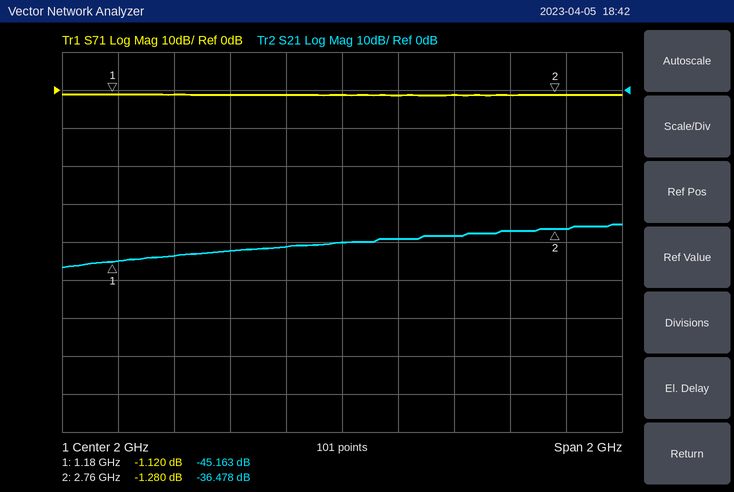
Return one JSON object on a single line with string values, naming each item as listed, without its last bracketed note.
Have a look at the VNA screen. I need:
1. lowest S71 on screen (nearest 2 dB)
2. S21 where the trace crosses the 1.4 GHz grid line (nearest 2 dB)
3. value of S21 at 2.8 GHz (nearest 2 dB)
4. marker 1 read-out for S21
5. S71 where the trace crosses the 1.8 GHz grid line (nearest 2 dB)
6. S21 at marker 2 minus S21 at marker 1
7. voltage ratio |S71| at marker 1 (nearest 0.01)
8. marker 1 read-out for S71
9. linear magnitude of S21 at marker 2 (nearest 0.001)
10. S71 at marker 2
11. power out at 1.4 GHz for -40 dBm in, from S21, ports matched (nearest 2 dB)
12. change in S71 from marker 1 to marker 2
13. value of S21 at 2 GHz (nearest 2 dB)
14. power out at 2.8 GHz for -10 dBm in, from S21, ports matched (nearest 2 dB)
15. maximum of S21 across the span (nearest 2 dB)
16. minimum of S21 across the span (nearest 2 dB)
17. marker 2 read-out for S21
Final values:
{"lowest S71 on screen": "-2 dB", "S21 where the trace crosses the 1.4 GHz grid line": "-44 dB", "value of S21 at 2.8 GHz": "-36 dB", "marker 1 read-out for S21": "-45.163 dB", "S71 where the trace crosses the 1.8 GHz grid line": "-2 dB", "S21 at marker 2 minus S21 at marker 1": "8.685 dB", "voltage ratio |S71| at marker 1": "0.88", "marker 1 read-out for S71": "-1.120 dB", "linear magnitude of S21 at marker 2": "0.015", "S71 at marker 2": "-1.280 dB", "power out at 1.4 GHz for -40 dBm in, from S21, ports matched": "-84 dBm", "change in S71 from marker 1 to marker 2": "-0.160 dB", "value of S21 at 2 GHz": "-40 dB", "power out at 2.8 GHz for -10 dBm in, from S21, ports matched": "-46 dBm", "maximum of S21 across the span": "-36 dB", "minimum of S21 across the span": "-46 dB", "marker 2 read-out for S21": "-36.478 dB"}
